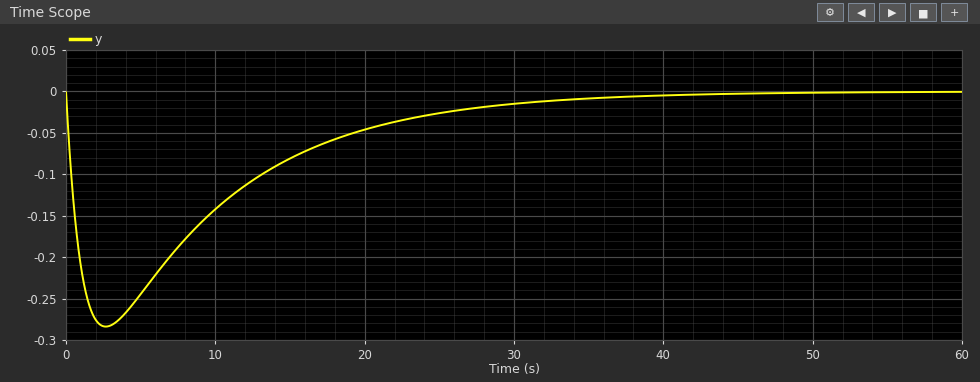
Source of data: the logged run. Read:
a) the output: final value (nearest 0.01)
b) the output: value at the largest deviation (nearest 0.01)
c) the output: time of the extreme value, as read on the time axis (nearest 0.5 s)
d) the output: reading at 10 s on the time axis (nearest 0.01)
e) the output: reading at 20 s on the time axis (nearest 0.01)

0.00
-0.28
2.5 s
-0.14
-0.05
